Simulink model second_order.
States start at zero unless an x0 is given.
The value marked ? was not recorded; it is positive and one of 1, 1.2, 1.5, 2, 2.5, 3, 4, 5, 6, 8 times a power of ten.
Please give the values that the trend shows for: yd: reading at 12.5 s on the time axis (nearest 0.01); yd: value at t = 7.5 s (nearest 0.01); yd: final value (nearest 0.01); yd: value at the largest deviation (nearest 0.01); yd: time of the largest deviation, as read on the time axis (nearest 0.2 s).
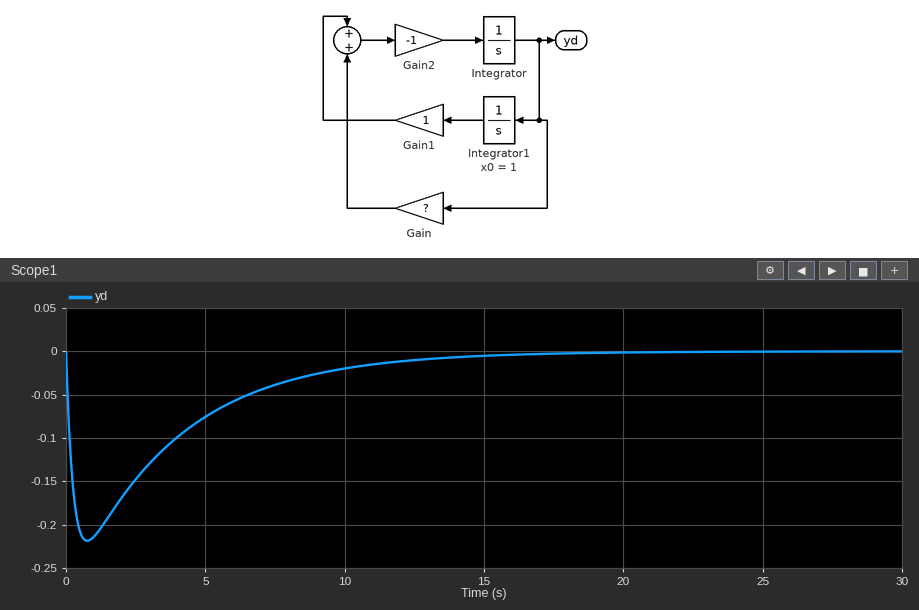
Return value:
-0.01
-0.04
0.00
-0.22
0.8 s
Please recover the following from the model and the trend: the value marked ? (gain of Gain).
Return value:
4
